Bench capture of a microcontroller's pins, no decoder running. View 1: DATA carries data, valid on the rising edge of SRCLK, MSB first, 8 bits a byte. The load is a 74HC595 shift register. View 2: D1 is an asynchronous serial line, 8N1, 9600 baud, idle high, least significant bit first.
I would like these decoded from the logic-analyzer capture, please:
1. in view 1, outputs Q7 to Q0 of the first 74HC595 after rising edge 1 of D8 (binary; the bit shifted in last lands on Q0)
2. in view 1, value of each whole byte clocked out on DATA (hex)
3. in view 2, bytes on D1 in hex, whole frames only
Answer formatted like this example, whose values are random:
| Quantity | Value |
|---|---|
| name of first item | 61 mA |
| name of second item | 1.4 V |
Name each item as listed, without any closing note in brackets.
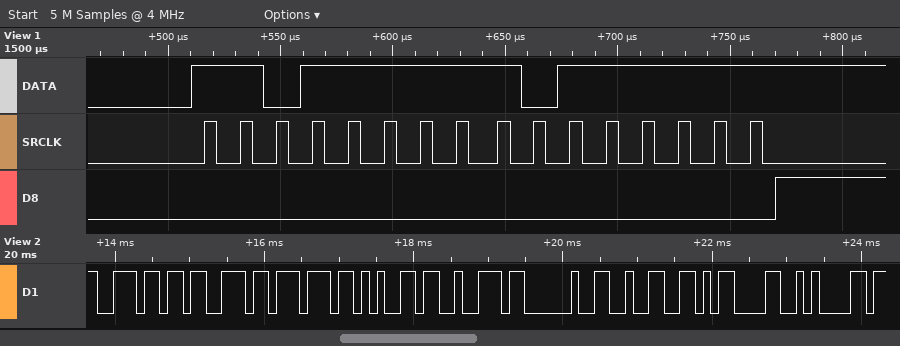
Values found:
| Quantity | Value |
|---|---|
| in view 1, outputs Q7 to Q0 of the first 74HC595 after rising edge 1 of D8 | 10111111 |
| in view 1, value of each whole byte clocked out on DATA | 0xDF 0xBF |
| in view 2, bytes on D1 in hex, whole frames only | 6E 73 77 65 72 20 32 0D 0A |
